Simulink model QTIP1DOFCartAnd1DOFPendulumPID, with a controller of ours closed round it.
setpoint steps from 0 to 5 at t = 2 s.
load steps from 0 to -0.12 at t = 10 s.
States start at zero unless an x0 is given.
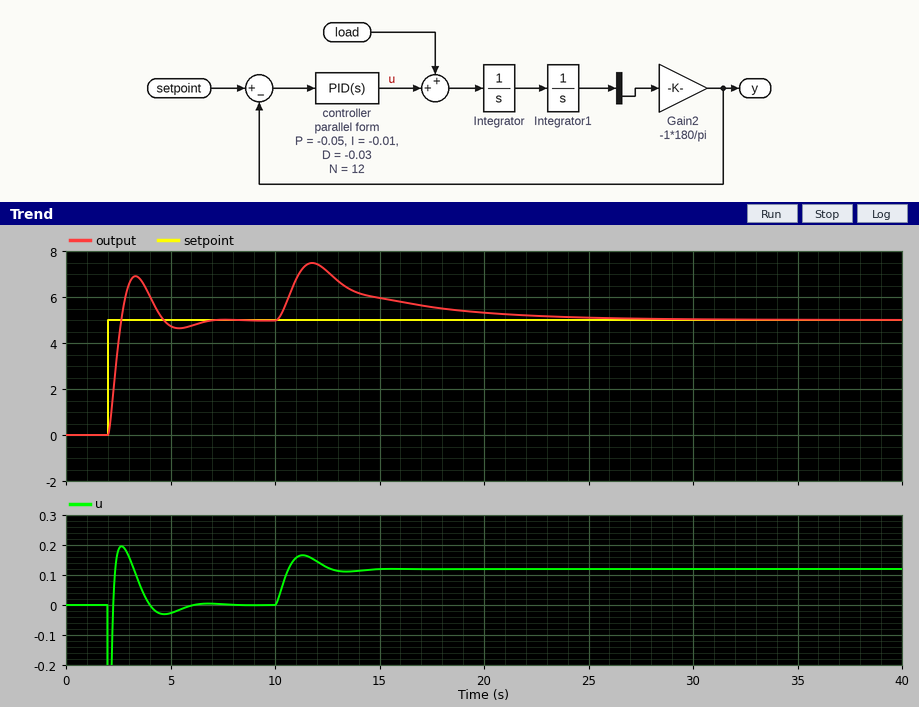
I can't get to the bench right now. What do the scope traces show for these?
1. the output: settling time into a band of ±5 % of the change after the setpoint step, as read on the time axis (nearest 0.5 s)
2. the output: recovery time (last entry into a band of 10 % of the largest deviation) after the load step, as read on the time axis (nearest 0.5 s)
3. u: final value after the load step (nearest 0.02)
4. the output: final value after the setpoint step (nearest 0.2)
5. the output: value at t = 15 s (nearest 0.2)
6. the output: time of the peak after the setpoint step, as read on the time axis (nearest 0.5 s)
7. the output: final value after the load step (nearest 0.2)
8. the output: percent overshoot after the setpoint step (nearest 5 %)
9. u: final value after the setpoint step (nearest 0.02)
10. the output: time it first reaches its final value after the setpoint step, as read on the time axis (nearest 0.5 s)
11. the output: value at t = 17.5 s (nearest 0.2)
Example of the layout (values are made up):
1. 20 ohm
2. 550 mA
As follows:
1. 6.0 s
2. 21.0 s
3. 0.12
4. 5.0
5. 6.0
6. 3.5 s
7. 5.0
8. 40 %
9. 0.00
10. 2.5 s
11. 5.6
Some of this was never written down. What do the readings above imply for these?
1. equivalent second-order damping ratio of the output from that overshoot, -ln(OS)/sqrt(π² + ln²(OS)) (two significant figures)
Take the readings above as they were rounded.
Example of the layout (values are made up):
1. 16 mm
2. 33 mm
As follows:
1. 0.28
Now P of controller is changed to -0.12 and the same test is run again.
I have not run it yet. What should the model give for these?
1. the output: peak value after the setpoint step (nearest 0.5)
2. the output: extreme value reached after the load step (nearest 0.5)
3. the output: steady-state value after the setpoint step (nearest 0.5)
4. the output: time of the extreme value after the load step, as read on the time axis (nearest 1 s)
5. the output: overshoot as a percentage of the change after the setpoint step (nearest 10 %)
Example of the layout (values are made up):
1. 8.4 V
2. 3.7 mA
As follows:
1. 7.5
2. 6.5
3. 5.0
4. 11 s
5. 50 %
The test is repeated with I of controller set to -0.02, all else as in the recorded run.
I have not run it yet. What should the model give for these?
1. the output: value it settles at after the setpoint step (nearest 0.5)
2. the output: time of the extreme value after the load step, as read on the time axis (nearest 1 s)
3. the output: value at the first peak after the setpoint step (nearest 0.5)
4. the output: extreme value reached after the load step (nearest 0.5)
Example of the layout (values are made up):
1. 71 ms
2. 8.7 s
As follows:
1. 5.0
2. 12 s
3. 7.0
4. 7.5
